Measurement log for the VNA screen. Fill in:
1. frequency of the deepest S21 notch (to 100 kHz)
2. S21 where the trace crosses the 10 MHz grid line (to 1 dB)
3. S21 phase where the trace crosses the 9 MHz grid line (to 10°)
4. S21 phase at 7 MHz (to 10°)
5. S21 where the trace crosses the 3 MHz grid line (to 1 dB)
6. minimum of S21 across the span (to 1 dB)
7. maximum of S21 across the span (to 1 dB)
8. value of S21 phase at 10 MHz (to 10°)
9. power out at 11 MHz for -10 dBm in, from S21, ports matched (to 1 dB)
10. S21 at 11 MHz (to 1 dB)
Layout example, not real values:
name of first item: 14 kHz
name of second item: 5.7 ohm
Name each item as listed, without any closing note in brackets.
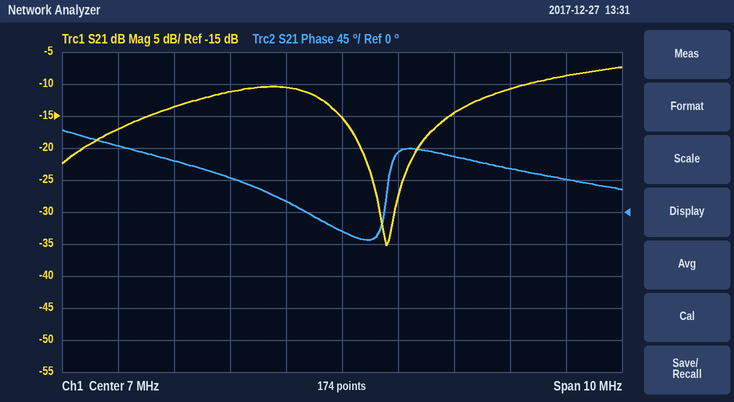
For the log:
frequency of the deepest S21 notch: 7.8 MHz
S21 where the trace crosses the 10 MHz grid line: -11 dB
S21 phase where the trace crosses the 9 MHz grid line: 80°
S21 phase at 7 MHz: -30°
S21 where the trace crosses the 3 MHz grid line: -17 dB
minimum of S21 across the span: -35 dB
maximum of S21 across the span: -7 dB
value of S21 phase at 10 MHz: 60°
power out at 11 MHz for -10 dBm in, from S21, ports matched: -19 dBm
S21 at 11 MHz: -9 dB
